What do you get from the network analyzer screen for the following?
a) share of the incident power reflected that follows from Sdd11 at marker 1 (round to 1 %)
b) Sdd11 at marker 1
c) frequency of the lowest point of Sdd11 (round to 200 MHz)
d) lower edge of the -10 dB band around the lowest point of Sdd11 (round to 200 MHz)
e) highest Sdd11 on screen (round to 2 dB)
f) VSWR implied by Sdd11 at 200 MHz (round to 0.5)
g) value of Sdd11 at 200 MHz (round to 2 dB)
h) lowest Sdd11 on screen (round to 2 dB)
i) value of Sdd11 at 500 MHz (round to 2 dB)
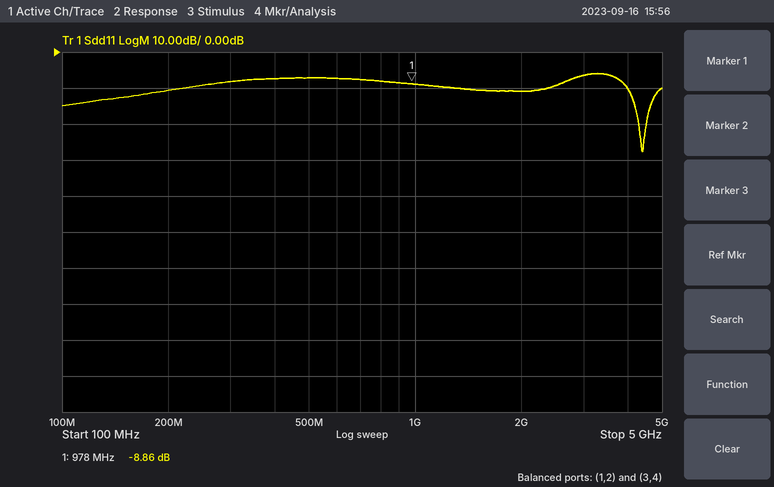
13 %
-8.86 dB
4.4 GHz
4.0 GHz
-6 dB
2.0
-10 dB
-28 dB
-8 dB
